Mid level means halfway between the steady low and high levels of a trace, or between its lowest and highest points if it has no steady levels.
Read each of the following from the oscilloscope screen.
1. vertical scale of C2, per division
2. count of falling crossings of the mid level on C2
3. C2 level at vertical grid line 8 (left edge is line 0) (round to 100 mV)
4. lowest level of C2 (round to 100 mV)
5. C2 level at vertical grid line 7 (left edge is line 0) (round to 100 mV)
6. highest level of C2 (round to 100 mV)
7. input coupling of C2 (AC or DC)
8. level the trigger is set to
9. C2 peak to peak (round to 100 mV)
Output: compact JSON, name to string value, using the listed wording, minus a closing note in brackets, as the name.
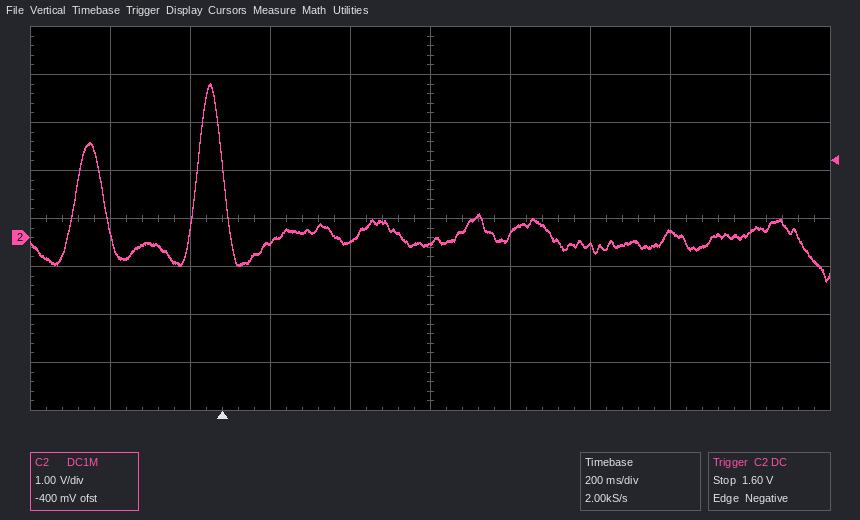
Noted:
{"vertical scale of C2, per division": "1 V", "count of falling crossings of the mid level on C2": "2", "C2 level at vertical grid line 8 (left edge is line 0)": "100 mV", "lowest level of C2": "-900 mV", "C2 level at vertical grid line 7 (left edge is line 0)": "-200 mV", "highest level of C2": "3.2 V", "input coupling of C2": "DC", "level the trigger is set to": "1.60 V", "C2 peak to peak": "4.1 V"}
